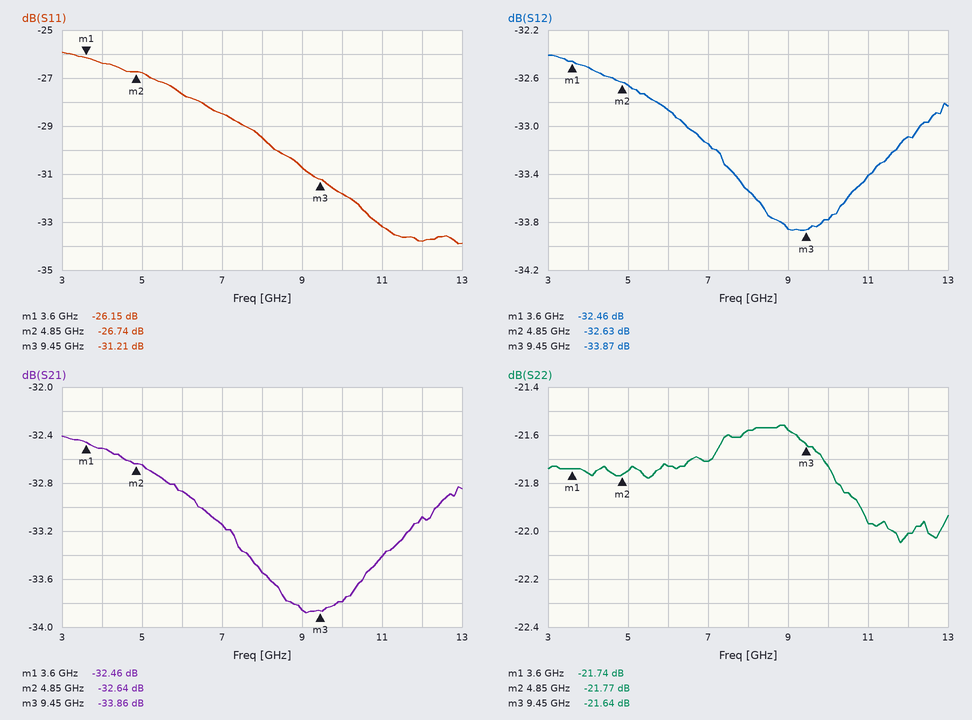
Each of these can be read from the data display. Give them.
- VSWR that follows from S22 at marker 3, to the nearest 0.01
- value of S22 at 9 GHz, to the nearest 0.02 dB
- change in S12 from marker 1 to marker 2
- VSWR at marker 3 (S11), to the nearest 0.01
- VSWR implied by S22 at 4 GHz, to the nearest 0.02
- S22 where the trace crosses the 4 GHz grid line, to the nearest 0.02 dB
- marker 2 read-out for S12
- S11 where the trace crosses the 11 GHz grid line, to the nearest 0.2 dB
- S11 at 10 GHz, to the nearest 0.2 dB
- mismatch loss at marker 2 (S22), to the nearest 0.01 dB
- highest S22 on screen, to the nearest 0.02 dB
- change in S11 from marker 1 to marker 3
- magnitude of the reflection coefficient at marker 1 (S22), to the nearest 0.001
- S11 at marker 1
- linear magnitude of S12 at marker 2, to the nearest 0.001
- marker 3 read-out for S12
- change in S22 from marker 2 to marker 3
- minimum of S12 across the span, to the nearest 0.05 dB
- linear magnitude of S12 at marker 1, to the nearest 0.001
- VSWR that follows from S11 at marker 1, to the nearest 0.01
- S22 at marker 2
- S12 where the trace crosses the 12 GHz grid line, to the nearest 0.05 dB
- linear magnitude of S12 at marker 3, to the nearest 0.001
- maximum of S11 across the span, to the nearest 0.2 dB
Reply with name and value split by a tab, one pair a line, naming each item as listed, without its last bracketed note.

VSWR that follows from S22 at marker 3, to the nearest 0.01	1.18
value of S22 at 9 GHz, to the nearest 0.02 dB	-21.58 dB
change in S12 from marker 1 to marker 2	-0.17 dB
VSWR at marker 3 (S11), to the nearest 0.01	1.06
VSWR implied by S22 at 4 GHz, to the nearest 0.02	1.18
S22 where the trace crosses the 4 GHz grid line, to the nearest 0.02 dB	-21.76 dB
marker 2 read-out for S12	-32.63 dB
S11 where the trace crosses the 11 GHz grid line, to the nearest 0.2 dB	-33.2 dB
S11 at 10 GHz, to the nearest 0.2 dB	-31.8 dB
mismatch loss at marker 2 (S22), to the nearest 0.01 dB	0.03 dB
highest S22 on screen, to the nearest 0.02 dB	-21.56 dB
change in S11 from marker 1 to marker 3	-5.06 dB
magnitude of the reflection coefficient at marker 1 (S22), to the nearest 0.001	0.082
S11 at marker 1	-26.15 dB
linear magnitude of S12 at marker 2, to the nearest 0.001	0.023
marker 3 read-out for S12	-33.87 dB
change in S22 from marker 2 to marker 3	0.13 dB
minimum of S12 across the span, to the nearest 0.05 dB	-33.85 dB
linear magnitude of S12 at marker 1, to the nearest 0.001	0.024
VSWR that follows from S11 at marker 1, to the nearest 0.01	1.10
S22 at marker 2	-21.77 dB
S12 where the trace crosses the 12 GHz grid line, to the nearest 0.05 dB	-33.10 dB
linear magnitude of S12 at marker 3, to the nearest 0.001	0.020
maximum of S11 across the span, to the nearest 0.2 dB	-26.0 dB
